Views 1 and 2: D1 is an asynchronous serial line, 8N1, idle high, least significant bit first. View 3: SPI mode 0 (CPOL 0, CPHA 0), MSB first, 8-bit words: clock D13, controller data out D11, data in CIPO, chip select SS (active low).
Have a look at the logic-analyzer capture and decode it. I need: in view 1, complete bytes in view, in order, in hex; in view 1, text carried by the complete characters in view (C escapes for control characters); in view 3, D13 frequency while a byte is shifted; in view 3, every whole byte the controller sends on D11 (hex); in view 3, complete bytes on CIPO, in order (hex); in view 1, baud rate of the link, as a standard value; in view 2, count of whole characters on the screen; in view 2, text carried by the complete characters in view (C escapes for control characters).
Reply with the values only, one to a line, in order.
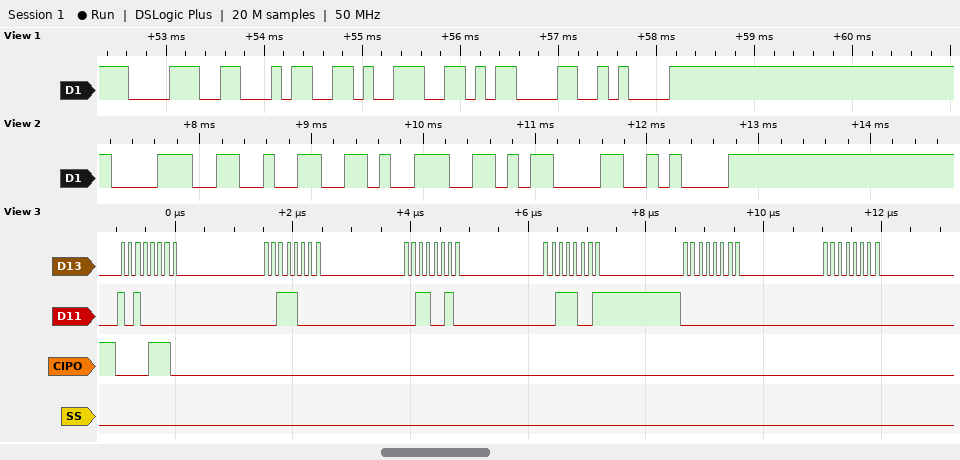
38 34 39 0D 0A
"849\r\n"
8 MHz
A0 38 32 39 00 00
0E 00 00 00 00 00
9600 baud
5
"829\r\n"
